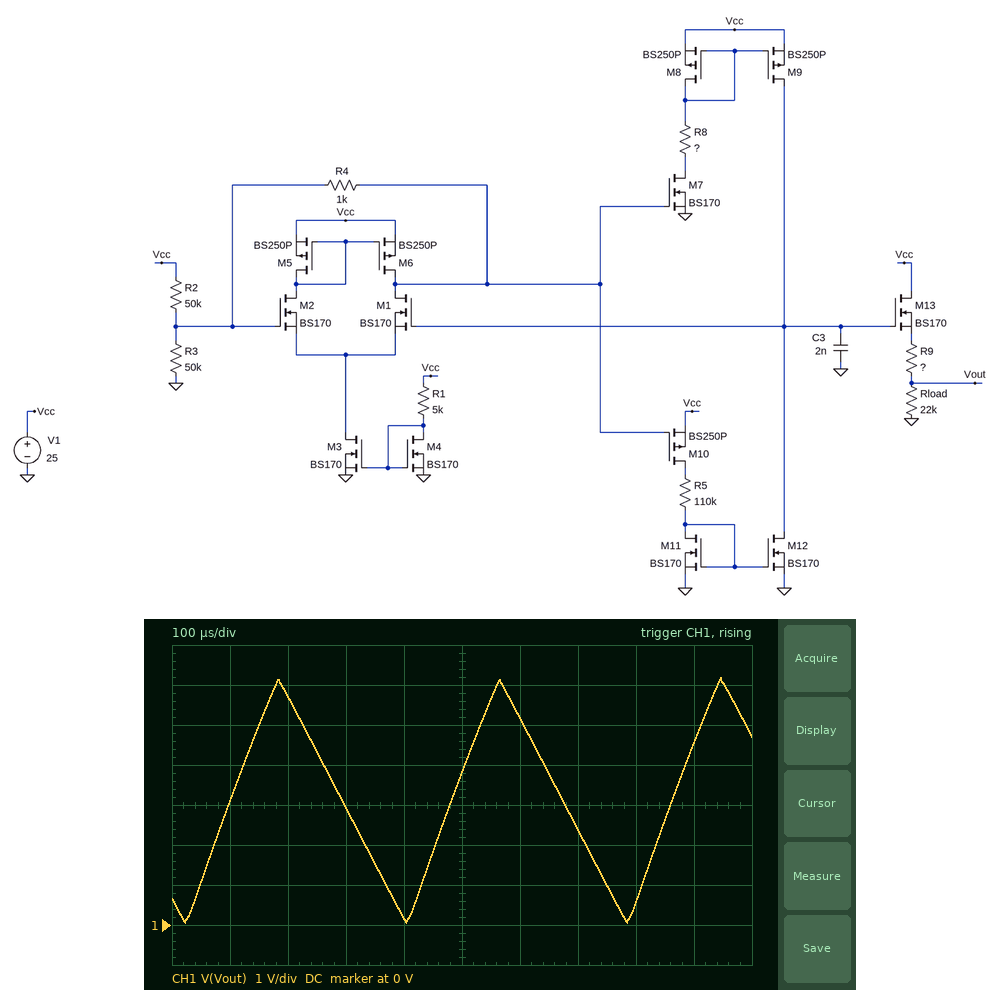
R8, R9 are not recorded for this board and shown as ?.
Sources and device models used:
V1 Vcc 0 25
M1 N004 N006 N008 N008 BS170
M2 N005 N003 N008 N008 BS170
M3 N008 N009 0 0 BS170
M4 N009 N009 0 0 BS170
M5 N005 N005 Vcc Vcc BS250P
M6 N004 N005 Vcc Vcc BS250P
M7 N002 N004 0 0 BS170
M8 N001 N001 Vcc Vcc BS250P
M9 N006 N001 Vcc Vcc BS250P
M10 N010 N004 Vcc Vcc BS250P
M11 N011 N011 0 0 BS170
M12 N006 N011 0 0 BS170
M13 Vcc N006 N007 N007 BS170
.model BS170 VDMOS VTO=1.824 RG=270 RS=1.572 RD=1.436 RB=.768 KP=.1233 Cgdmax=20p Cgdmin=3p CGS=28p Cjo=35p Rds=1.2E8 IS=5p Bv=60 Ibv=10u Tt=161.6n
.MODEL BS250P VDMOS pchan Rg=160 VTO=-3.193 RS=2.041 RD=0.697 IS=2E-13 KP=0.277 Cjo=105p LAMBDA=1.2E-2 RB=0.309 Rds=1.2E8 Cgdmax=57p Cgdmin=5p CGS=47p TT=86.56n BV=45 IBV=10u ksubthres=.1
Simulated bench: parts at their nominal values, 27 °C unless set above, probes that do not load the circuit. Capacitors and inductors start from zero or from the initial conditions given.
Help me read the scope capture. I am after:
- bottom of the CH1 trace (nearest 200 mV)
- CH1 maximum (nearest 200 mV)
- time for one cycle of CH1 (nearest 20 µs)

0 V
6.2 V
380 µs
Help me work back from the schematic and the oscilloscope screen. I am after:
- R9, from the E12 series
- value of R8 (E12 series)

56 kΩ
82 kΩ
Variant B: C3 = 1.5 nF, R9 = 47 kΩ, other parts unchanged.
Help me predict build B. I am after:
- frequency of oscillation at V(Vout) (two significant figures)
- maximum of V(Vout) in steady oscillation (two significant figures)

3.4 kHz
7.0 V
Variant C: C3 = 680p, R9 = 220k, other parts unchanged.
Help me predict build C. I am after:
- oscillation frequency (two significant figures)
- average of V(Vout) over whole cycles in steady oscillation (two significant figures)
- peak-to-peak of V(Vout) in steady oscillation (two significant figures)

6.8 kHz
1.0 V
2.0 V
